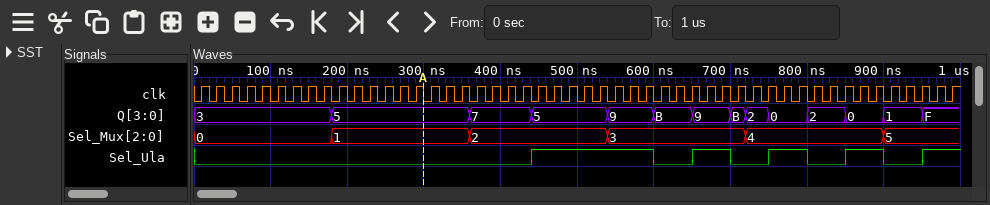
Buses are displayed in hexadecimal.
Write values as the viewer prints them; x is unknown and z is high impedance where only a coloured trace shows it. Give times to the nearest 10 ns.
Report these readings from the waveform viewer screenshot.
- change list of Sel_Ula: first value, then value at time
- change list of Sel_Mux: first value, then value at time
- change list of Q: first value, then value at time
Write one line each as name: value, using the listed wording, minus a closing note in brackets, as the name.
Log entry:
change list of Sel_Ula: first value, then value at time: 0, 1 at 440 ns, 0 at 600 ns, 1 at 650 ns, 0 at 700 ns, 1 at 750 ns, 0 at 800 ns, 1 at 850 ns, 0 at 900 ns, 1 at 950 ns
change list of Sel_Mux: first value, then value at time: 0, 1 at 180 ns, 2 at 360 ns, 3 at 540 ns, 4 at 720 ns, 5 at 900 ns
change list of Q: first value, then value at time: 3, 5 at 180 ns, 7 at 360 ns, 5 at 440 ns, 9 at 540 ns, B at 600 ns, 9 at 650 ns, B at 700 ns, 2 at 720 ns, 0 at 750 ns, 2 at 800 ns, 0 at 850 ns, 1 at 900 ns, F at 950 ns
